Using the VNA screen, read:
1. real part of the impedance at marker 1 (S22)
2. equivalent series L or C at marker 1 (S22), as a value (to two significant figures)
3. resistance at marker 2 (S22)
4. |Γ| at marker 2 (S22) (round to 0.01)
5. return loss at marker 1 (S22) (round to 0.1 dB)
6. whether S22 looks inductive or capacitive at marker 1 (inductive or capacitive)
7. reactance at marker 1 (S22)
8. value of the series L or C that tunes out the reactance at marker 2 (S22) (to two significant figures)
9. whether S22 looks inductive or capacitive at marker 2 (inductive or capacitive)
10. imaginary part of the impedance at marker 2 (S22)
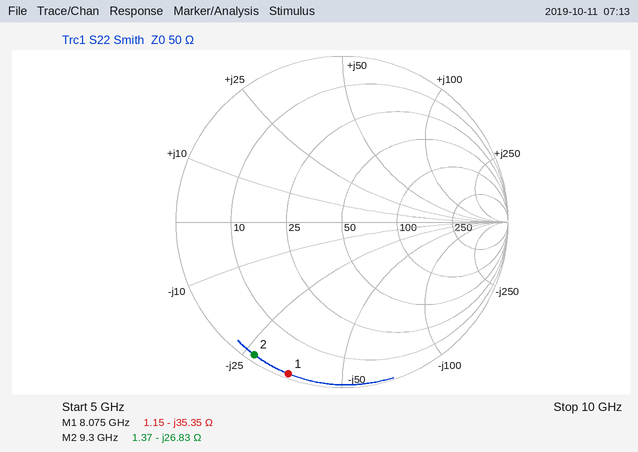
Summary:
1.15 Ω
560 fF
1.37 Ω
0.96
0.3 dB
capacitive
-35.35 Ω
460 pH
capacitive
-26.83 Ω
